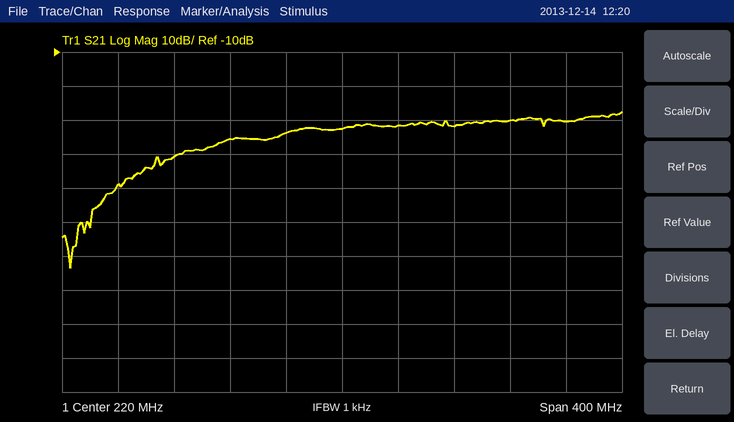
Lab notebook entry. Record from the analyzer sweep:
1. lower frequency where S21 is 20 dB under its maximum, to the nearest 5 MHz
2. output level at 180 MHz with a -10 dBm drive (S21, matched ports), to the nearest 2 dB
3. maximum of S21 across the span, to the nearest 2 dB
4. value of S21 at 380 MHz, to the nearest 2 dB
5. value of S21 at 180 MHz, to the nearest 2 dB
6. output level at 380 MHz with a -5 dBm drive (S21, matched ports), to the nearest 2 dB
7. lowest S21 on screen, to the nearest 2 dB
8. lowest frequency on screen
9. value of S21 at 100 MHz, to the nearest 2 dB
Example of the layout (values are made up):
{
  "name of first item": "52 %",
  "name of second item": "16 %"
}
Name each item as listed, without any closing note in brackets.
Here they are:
{
  "lower frequency where S21 is 20 dB under its maximum, to the nearest 5 MHz": "65 MHz",
  "output level at 180 MHz with a -10 dBm drive (S21, matched ports), to the nearest 2 dB": "-44 dBm",
  "maximum of S21 across the span, to the nearest 2 dB": "-28 dB",
  "value of S21 at 380 MHz, to the nearest 2 dB": "-30 dB",
  "value of S21 at 180 MHz, to the nearest 2 dB": "-34 dB",
  "output level at 380 MHz with a -5 dBm drive (S21, matched ports), to the nearest 2 dB": "-36 dBm",
  "lowest S21 on screen, to the nearest 2 dB": "-74 dB",
  "lowest frequency on screen": "20 MHz",
  "value of S21 at 100 MHz, to the nearest 2 dB": "-40 dB"
}
